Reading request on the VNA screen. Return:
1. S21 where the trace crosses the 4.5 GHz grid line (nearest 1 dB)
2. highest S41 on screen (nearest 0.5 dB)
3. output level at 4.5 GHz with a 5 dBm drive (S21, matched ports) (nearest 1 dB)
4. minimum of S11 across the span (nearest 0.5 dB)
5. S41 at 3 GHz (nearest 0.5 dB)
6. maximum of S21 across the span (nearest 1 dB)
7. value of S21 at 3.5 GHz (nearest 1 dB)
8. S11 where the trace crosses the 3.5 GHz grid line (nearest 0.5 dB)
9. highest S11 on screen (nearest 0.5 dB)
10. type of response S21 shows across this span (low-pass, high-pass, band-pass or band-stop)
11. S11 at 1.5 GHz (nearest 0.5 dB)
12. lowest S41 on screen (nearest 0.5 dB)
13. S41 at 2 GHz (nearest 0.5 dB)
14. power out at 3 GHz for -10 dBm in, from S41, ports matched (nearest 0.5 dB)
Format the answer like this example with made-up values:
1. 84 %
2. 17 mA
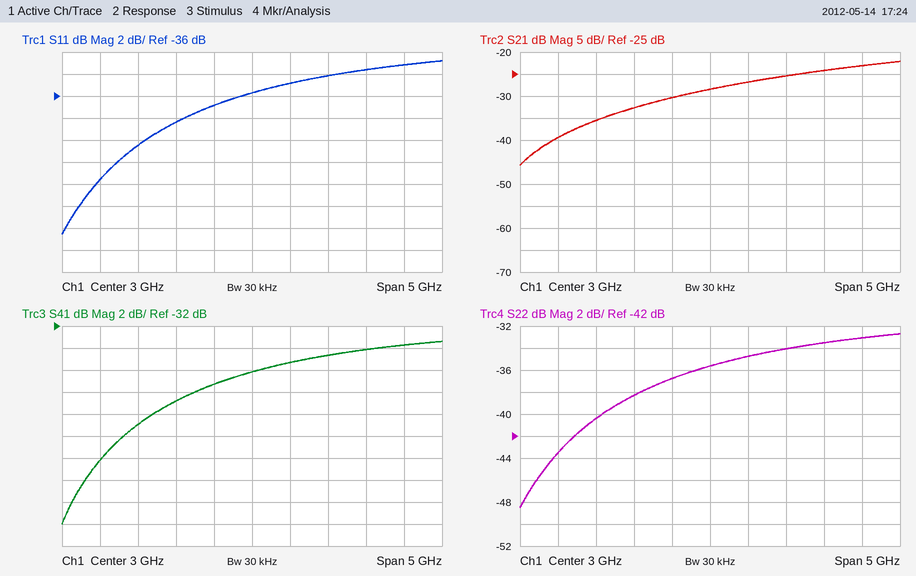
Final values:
1. -24 dB
2. -33.5 dB
3. -19 dBm
4. -48.5 dB
5. -36.0 dB
6. -22 dB
7. -27 dB
8. -35.0 dB
9. -33.0 dB
10. high-pass
11. -40.5 dB
12. -50.0 dB
13. -39.0 dB
14. -46.0 dBm
